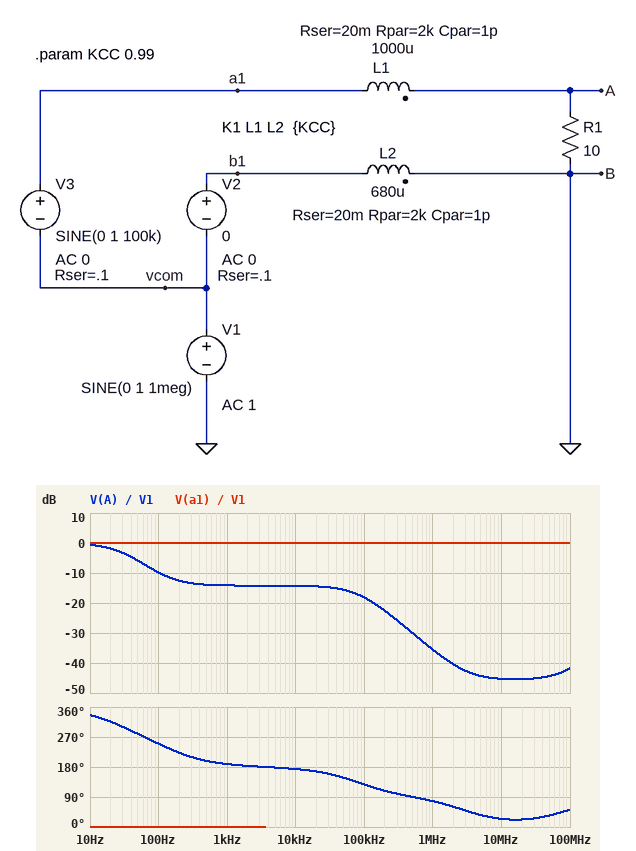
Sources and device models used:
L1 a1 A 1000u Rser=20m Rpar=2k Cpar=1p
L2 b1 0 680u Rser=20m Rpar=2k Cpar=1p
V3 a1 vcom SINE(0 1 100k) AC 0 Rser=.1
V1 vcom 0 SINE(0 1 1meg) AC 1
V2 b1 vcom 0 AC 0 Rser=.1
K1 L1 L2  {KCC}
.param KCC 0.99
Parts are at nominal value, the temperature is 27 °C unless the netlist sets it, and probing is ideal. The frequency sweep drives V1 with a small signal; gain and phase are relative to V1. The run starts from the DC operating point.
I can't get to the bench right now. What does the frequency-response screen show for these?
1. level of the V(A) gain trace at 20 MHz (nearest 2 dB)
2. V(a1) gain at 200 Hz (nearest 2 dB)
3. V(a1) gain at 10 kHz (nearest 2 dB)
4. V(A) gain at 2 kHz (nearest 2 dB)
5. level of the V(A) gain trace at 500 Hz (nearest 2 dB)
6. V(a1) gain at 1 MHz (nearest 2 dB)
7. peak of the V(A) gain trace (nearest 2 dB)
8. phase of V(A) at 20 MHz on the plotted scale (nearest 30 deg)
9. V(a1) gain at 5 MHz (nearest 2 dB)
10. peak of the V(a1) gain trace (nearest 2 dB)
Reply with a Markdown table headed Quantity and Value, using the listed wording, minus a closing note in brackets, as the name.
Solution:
| Quantity | Value |
|---|---|
| level of the V(A) gain trace at 20 MHz | -46 dB |
| V(a1) gain at 200 Hz | 0 dB |
| V(a1) gain at 10 kHz | 0 dB |
| V(A) gain at 2 kHz | -14 dB |
| level of the V(A) gain trace at 500 Hz | -14 dB |
| V(a1) gain at 1 MHz | 0 dB |
| peak of the V(A) gain trace | 0 dB |
| phase of V(A) at 20 MHz on the plotted scale | 30 deg |
| V(a1) gain at 5 MHz | 0 dB |
| peak of the V(a1) gain trace | 0 dB |
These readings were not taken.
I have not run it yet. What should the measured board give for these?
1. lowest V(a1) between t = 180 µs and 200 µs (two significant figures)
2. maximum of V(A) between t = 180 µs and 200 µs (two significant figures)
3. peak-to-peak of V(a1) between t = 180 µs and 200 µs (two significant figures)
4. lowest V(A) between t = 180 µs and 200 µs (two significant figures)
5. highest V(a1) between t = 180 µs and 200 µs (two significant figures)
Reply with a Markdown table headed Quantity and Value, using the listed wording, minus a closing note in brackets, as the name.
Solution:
| Quantity | Value |
|---|---|
| lowest V(a1) between t = 180 µs and 200 µs | -2.0 V |
| maximum of V(A) between t = 180 µs and 200 µs | 630 mV |
| peak-to-peak of V(a1) between t = 180 µs and 200 µs | 4.0 V |
| lowest V(A) between t = 180 µs and 200 µs | -620 mV |
| highest V(a1) between t = 180 µs and 200 µs | 2.0 V |
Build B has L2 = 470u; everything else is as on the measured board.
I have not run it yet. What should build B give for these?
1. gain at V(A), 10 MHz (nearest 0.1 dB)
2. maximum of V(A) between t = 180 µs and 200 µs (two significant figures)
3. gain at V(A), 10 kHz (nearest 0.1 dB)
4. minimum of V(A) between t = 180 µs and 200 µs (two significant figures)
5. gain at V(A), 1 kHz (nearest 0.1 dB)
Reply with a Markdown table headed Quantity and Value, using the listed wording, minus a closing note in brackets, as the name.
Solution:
| Quantity | Value |
|---|---|
| gain at V(A), 10 MHz | -43.8 dB |
| maximum of V(A) between t = 180 µs and 200 µs | 650 mV |
| gain at V(A), 10 kHz | -7.4 dB |
| minimum of V(A) between t = 180 µs and 200 µs | -630 mV |
| gain at V(A), 1 kHz | -7.3 dB |
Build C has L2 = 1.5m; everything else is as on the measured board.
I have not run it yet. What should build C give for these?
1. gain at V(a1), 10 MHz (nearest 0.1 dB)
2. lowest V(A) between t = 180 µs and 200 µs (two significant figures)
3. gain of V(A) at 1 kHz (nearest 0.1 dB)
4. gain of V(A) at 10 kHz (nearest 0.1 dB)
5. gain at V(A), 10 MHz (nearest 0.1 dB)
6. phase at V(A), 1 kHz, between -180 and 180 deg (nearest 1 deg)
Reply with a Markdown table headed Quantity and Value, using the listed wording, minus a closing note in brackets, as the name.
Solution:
| Quantity | Value |
|---|---|
| gain at V(a1), 10 MHz | 0 dB |
| lowest V(A) between t = 180 µs and 200 µs | -630 mV |
| gain of V(A) at 1 kHz | -14.5 dB |
| gain of V(A) at 10 kHz | -14.6 dB |
| gain at V(A), 10 MHz | -45.9 dB |
| phase at V(A), 1 kHz, between -180 and 180 deg | -4 deg |
